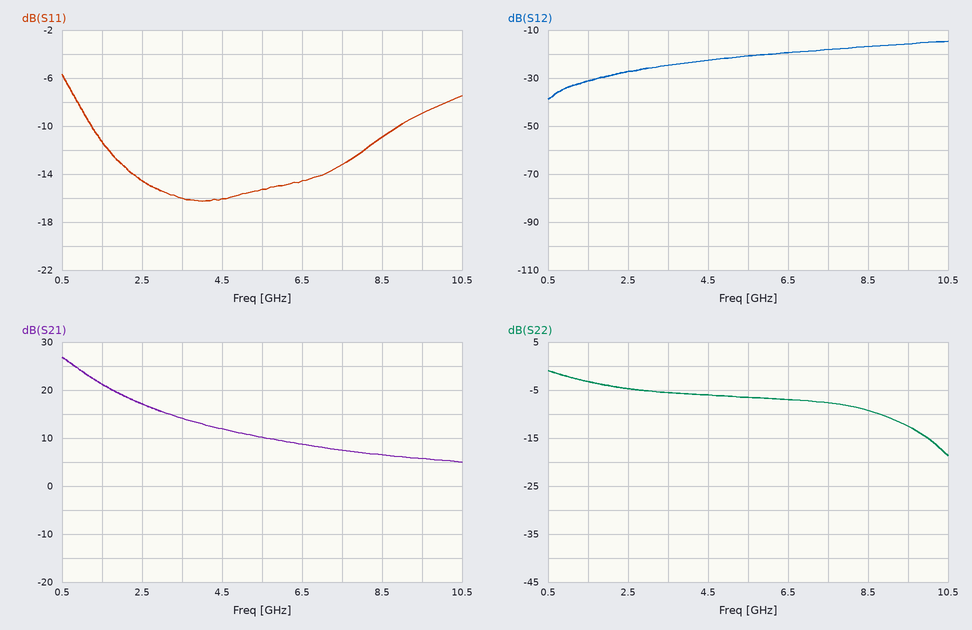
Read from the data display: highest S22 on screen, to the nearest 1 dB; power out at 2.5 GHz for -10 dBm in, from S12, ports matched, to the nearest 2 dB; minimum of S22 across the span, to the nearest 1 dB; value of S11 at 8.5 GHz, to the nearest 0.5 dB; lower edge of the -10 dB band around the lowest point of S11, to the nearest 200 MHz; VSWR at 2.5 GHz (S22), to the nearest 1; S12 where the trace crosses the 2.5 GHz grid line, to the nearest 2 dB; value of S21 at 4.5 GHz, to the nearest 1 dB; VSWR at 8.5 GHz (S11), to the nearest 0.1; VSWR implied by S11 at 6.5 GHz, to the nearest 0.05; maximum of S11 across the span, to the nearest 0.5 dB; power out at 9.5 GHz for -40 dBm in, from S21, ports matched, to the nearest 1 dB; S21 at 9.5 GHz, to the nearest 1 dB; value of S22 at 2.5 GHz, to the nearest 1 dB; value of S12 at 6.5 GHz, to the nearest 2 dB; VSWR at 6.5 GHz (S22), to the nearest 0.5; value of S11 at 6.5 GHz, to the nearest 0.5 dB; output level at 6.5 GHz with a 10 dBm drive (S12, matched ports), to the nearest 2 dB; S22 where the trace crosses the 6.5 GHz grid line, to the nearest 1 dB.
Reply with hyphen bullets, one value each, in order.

- -1 dB
- -38 dBm
- -19 dB
- -11.0 dB
- 1.2 GHz
- 4
- -28 dB
- 12 dB
- 1.8
- 1.45
- -5.5 dB
- -34 dBm
- 6 dB
- -5 dB
- -20 dB
- 2.5
- -14.5 dB
- -10 dBm
- -7 dB
